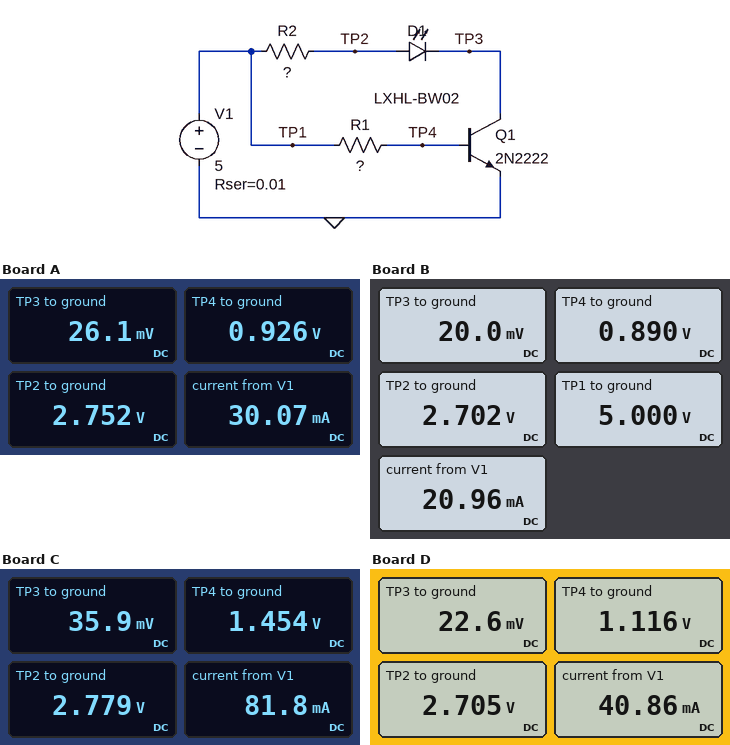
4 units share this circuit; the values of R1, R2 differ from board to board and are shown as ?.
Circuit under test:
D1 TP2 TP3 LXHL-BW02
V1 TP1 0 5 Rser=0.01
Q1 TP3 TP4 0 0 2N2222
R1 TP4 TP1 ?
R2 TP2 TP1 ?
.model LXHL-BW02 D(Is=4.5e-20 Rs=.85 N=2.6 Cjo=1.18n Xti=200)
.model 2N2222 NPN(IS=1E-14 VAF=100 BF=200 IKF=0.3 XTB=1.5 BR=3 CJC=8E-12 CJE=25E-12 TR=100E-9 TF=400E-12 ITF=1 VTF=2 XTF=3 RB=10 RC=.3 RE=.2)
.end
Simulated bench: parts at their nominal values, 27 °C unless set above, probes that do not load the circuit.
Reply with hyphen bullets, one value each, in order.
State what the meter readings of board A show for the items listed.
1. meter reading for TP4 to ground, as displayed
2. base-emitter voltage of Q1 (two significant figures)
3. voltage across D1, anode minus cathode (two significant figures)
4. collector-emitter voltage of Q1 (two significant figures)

- 0.926 V
- 930 mV
- 2.7 V
- 26 mV
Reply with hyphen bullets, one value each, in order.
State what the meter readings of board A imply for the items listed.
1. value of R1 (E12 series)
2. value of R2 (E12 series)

- 270 Ω
- 150 Ω
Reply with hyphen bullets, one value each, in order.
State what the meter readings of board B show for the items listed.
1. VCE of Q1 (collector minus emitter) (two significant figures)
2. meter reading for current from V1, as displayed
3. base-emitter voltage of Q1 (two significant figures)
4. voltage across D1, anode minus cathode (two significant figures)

- 20 mV
- 20.96 mA
- 890 mV
- 2.7 V
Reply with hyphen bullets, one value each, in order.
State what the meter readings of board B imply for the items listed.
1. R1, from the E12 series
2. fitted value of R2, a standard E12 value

- 330 Ω
- 270 Ω
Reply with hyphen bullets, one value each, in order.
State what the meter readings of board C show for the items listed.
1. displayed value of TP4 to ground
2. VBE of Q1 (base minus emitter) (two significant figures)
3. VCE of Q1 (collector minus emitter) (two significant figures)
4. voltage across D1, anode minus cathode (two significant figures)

- 1.454 V
- 1.5 V
- 36 mV
- 2.7 V
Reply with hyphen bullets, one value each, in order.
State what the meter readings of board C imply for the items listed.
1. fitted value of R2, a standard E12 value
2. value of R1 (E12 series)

- 120 Ω
- 56 Ω
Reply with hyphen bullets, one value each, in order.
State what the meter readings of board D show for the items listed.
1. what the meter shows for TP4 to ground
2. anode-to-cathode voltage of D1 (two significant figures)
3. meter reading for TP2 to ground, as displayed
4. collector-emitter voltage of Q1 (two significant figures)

- 1.116 V
- 2.7 V
- 2.705 V
- 23 mV
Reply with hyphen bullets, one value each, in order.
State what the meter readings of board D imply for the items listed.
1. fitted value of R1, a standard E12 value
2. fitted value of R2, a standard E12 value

- 120 Ω
- 270 Ω
